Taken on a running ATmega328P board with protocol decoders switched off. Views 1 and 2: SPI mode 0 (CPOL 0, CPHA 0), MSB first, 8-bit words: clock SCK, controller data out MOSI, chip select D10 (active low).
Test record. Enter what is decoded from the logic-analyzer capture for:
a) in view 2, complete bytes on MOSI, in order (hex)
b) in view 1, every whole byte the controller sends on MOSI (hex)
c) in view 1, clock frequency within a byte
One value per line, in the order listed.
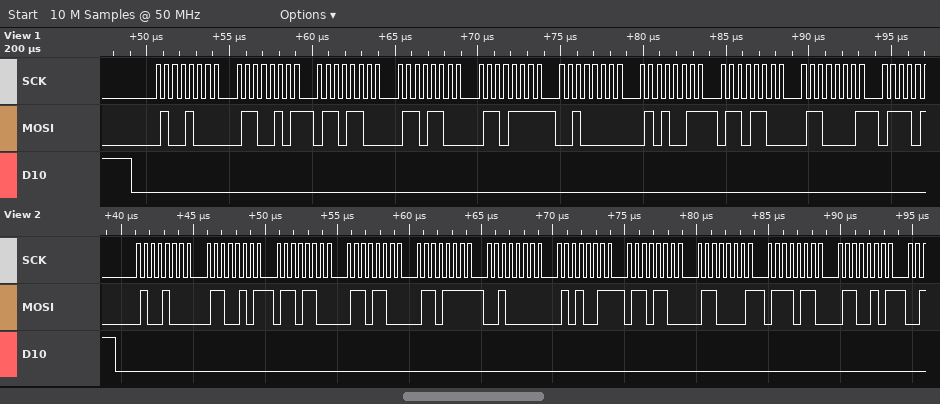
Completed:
48 65 6C 6C 6F 20 53 6C 61 76 65
0x48 0x65 0x6C 0x6C 0x6F 0x20 0x53 0x6C 0x61
2 MHz
